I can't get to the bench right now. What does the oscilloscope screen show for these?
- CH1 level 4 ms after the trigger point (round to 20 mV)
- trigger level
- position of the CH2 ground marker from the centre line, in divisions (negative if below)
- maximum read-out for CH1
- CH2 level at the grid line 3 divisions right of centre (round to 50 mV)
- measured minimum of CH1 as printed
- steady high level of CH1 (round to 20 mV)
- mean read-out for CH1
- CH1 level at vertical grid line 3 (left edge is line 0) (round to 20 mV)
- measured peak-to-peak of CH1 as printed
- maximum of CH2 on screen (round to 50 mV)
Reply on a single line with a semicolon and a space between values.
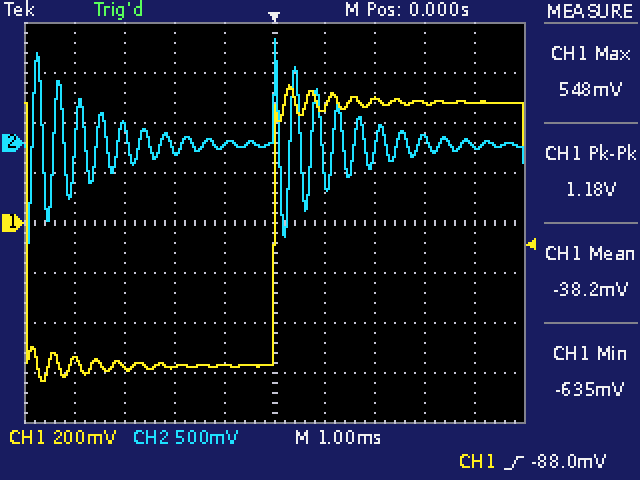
480 mV; -88.0 mV; +1.6 div; 548 mV; 50 mV; -635 mV; 480 mV; -38.2 mV; -580 mV; 1.18 V; 1.05 V
